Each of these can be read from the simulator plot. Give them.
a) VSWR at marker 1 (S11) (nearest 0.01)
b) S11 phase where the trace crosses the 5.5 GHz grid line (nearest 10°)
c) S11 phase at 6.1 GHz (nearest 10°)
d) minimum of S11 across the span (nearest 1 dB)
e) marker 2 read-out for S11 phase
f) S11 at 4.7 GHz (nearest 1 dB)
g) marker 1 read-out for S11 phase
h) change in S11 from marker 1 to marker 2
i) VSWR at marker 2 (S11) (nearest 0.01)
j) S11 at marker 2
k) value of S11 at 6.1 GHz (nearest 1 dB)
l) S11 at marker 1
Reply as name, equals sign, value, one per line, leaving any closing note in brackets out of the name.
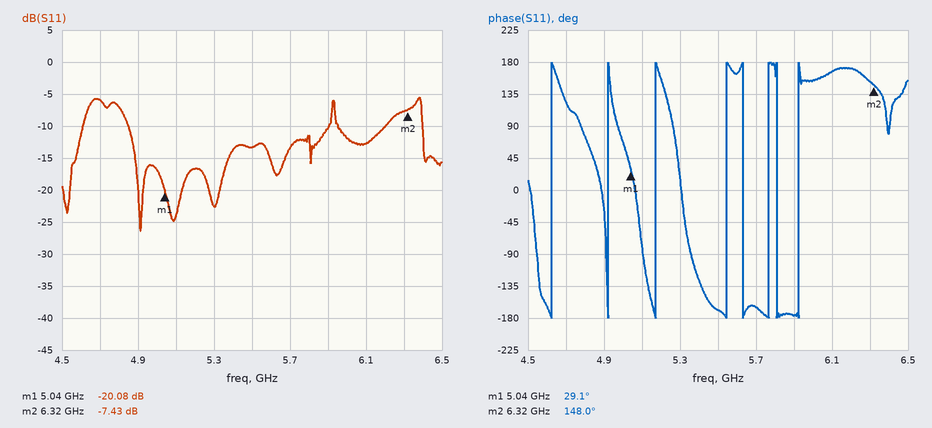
VSWR at marker 1 (S11) = 1.22
S11 phase where the trace crosses the 5.5 GHz grid line = -170°
S11 phase at 6.1 GHz = 170°
minimum of S11 across the span = -26 dB
marker 2 read-out for S11 phase = 148.0°
S11 at 4.7 GHz = -6 dB
marker 1 read-out for S11 phase = 29.1°
change in S11 from marker 1 to marker 2 = 12.65 dB
VSWR at marker 2 (S11) = 2.48
S11 at marker 2 = -7.43 dB
value of S11 at 6.1 GHz = -13 dB
S11 at marker 1 = -20.08 dB
